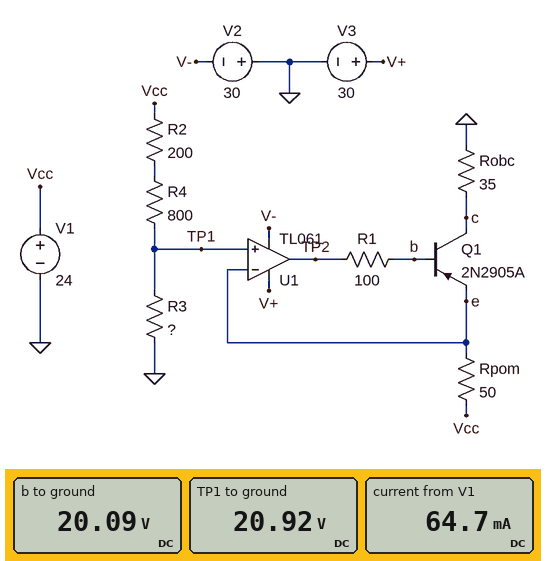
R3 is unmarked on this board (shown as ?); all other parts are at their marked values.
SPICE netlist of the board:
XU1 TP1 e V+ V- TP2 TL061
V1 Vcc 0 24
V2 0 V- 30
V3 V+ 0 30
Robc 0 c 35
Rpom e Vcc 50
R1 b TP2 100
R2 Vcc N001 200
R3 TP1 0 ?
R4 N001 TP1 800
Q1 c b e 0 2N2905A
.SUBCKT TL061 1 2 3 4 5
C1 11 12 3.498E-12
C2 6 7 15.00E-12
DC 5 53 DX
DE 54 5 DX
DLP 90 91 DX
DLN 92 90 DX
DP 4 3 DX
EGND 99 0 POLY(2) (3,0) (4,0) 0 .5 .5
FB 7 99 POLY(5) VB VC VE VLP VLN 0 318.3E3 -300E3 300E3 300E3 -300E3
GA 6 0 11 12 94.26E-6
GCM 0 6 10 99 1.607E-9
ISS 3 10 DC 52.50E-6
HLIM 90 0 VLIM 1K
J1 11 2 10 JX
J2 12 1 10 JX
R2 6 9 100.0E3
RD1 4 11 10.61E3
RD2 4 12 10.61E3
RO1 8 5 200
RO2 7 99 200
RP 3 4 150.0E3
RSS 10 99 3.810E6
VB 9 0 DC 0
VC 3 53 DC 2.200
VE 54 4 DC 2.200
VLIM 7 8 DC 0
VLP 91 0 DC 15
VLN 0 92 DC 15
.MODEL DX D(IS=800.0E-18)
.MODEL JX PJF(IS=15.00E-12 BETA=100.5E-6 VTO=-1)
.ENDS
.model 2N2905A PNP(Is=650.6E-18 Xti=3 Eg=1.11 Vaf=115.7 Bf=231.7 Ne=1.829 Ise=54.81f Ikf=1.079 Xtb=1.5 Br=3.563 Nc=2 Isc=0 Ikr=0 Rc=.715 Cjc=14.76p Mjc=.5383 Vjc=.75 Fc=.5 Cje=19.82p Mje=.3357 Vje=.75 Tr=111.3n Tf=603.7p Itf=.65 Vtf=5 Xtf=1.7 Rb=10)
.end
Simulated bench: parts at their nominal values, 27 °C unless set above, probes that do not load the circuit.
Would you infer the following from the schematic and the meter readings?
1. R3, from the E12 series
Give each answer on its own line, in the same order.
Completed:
6.8 kΩ
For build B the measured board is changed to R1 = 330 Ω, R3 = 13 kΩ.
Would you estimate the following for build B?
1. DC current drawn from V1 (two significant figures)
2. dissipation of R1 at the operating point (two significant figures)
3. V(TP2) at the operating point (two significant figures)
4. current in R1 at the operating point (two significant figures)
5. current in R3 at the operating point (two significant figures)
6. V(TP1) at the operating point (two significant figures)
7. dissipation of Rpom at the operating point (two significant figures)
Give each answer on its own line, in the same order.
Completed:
36 mA
5.6 µW
21 V
130 µA
1.7 mA
22 V
59 mW
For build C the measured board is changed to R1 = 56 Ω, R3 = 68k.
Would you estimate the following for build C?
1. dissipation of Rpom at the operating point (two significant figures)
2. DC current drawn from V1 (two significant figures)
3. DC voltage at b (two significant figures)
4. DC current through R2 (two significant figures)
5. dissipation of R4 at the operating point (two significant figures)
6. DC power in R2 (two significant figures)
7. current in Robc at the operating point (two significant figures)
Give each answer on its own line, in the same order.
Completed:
2.5 mW
7.4 mA
23 V
350 µA
97 µW
24 µW
7.0 mA
